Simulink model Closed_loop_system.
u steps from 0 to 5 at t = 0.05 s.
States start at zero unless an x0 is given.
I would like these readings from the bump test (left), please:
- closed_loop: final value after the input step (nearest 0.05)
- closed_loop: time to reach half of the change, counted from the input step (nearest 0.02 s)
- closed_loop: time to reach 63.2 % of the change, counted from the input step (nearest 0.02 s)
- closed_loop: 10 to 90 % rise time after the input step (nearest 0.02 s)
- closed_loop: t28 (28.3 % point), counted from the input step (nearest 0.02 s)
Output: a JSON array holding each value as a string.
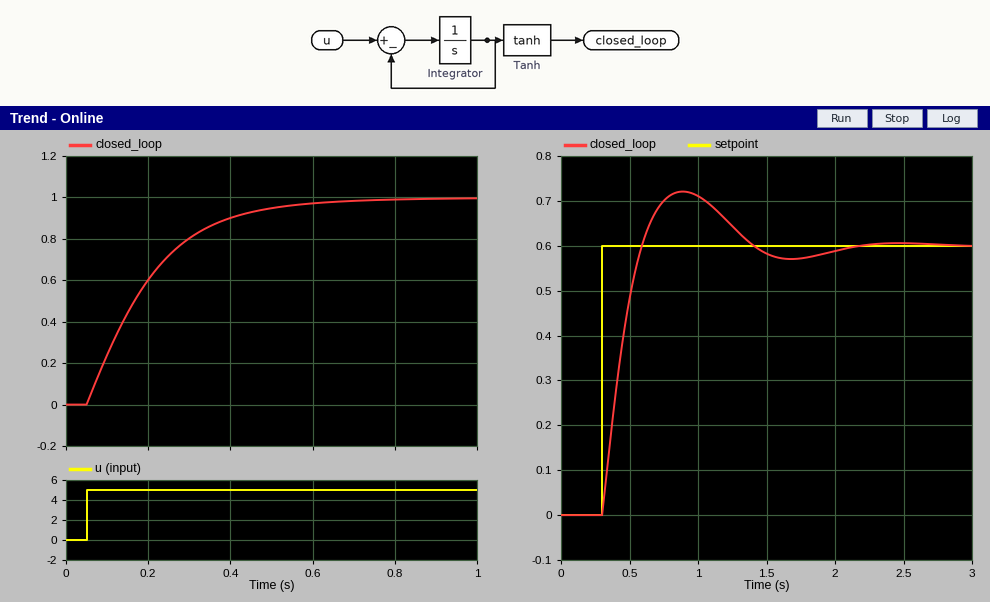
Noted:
["1.00", "0.12 s", "0.16 s", "0.32 s", "0.06 s"]
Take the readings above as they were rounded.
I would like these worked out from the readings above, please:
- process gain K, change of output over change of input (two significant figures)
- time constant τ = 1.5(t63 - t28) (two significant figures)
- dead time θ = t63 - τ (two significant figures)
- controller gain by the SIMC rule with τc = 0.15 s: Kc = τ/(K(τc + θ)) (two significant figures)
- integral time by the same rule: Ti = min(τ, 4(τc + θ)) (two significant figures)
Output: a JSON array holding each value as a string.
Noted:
["0.20", "0.15 s", "0.010 s", "4.7", "0.15 s"]
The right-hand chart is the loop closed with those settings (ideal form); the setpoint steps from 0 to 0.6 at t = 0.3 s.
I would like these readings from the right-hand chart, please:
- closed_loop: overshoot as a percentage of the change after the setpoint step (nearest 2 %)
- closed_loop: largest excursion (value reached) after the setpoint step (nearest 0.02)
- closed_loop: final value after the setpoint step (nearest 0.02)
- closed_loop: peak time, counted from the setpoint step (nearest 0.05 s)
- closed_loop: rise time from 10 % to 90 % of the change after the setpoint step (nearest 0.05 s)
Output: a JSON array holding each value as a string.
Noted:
["20 %", "0.72", "0.60", "0.60 s", "0.20 s"]
